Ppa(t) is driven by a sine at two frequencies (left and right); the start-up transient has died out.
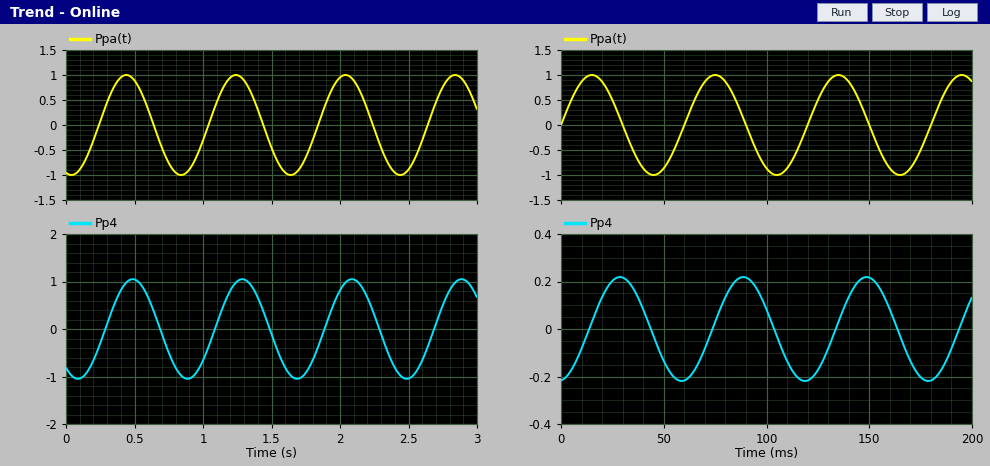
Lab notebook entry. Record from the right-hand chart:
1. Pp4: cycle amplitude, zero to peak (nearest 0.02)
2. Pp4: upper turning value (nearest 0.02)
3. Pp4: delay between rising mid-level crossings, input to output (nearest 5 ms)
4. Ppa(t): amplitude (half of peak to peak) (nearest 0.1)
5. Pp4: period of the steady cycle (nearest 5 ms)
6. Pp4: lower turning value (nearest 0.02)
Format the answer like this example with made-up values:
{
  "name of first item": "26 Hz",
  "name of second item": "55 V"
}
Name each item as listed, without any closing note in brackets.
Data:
{
  "Pp4: cycle amplitude, zero to peak": "0.22",
  "Pp4: upper turning value": "0.22",
  "Pp4: delay between rising mid-level crossings, input to output": "15 ms",
  "Ppa(t): amplitude (half of peak to peak)": "1.0",
  "Pp4: period of the steady cycle": "60 ms",
  "Pp4: lower turning value": "-0.22"
}
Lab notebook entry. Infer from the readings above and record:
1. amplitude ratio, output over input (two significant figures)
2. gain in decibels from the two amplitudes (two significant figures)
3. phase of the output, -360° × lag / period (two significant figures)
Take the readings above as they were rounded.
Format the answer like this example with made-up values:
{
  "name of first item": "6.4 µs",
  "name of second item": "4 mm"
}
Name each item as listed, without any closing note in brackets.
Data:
{
  "amplitude ratio, output over input": "0.22",
  "gain in decibels from the two amplitudes": "-13 dB",
  "phase of the output, -360° × lag / period": "-90°"
}
